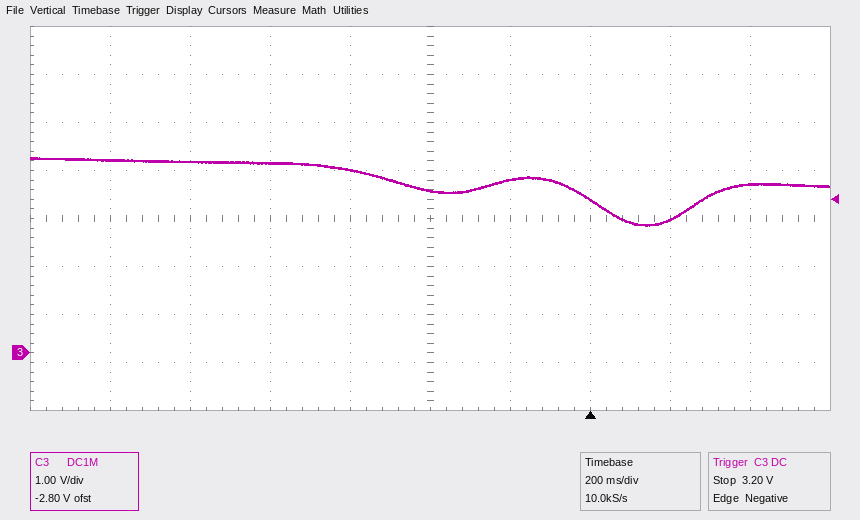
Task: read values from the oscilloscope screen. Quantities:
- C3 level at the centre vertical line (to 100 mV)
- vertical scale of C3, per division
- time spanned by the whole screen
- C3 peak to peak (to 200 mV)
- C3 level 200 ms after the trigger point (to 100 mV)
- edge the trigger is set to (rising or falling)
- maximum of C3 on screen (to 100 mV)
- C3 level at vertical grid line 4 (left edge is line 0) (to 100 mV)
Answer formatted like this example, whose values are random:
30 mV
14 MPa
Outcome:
3.4 V
1 V
2 s
1.4 V
2.8 V
falling
4.1 V
3.8 V
